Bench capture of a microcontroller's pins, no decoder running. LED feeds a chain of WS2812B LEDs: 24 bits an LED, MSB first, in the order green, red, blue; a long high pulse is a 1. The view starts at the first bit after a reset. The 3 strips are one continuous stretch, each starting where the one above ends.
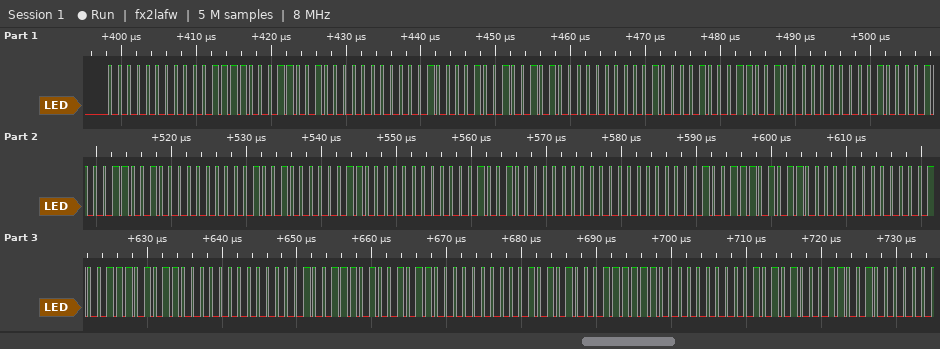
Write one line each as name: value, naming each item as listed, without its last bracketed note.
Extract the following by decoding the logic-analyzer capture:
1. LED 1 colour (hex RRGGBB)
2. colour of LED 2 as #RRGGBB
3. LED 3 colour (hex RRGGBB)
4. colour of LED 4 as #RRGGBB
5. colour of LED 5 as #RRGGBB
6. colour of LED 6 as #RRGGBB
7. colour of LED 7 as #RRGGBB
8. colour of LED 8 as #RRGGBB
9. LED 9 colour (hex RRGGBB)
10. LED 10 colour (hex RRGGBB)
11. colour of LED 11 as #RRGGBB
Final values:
LED 1 colour: #1E0032
colour of LED 2 as #RRGGBB: #210025
LED 3 colour: #210019
colour of LED 4 as #RRGGBB: #210019
colour of LED 5 as #RRGGBB: #24000C
colour of LED 6 as #RRGGBB: #240000
colour of LED 7 as #RRGGBB: #270058
colour of LED 8 as #RRGGBB: #270058
LED 9 colour: #27004B
LED 10 colour: #2A003F
colour of LED 11 as #RRGGBB: #2A0032
